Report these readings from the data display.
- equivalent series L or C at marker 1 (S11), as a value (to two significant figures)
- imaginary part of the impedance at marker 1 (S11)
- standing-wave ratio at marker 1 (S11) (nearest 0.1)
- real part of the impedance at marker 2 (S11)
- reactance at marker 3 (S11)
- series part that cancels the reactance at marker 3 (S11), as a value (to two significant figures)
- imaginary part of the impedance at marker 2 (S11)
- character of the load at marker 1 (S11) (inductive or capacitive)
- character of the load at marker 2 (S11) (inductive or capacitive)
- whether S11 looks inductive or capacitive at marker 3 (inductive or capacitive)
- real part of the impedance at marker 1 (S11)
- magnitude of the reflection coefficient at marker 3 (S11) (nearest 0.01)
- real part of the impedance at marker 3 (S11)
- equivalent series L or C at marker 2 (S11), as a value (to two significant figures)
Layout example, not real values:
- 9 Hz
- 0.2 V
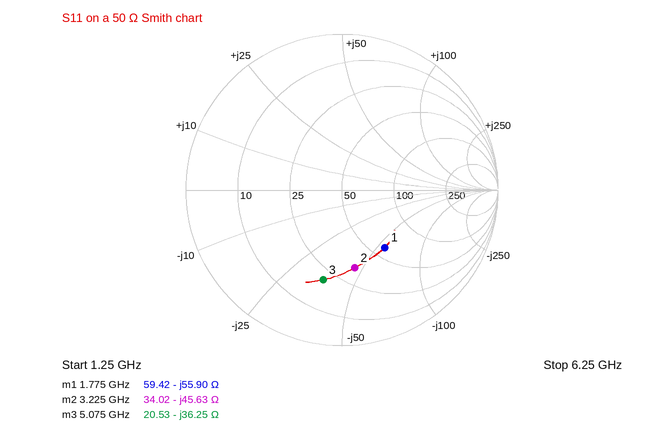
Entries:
- 1.6 pF
- -55.90 Ω
- 2.7
- 34.02 Ω
- -36.25 Ω
- 1.1 nH
- -45.63 Ω
- capacitive
- capacitive
- capacitive
- 59.42 Ω
- 0.59
- 20.53 Ω
- 1.1 pF
